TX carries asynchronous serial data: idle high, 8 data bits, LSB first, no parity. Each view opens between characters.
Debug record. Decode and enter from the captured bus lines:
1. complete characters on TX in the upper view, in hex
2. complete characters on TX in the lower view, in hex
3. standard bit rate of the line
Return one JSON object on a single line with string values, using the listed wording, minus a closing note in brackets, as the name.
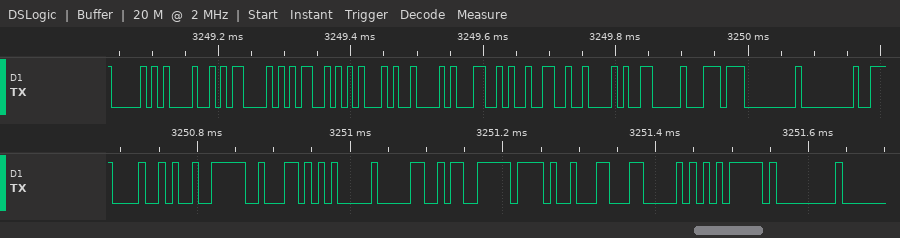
{"complete characters on TX in the upper view, in hex": "50, 48, 43, 4D, 45, 42, 4C, 32, 42, 06, DC, 00, 00", "complete characters on TX in the lower view, in hex": "48, F2, 62, 05, 30, F3, 2F, 8C, 50, 7D, 00", "standard bit rate of the line": "115200 baud"}
